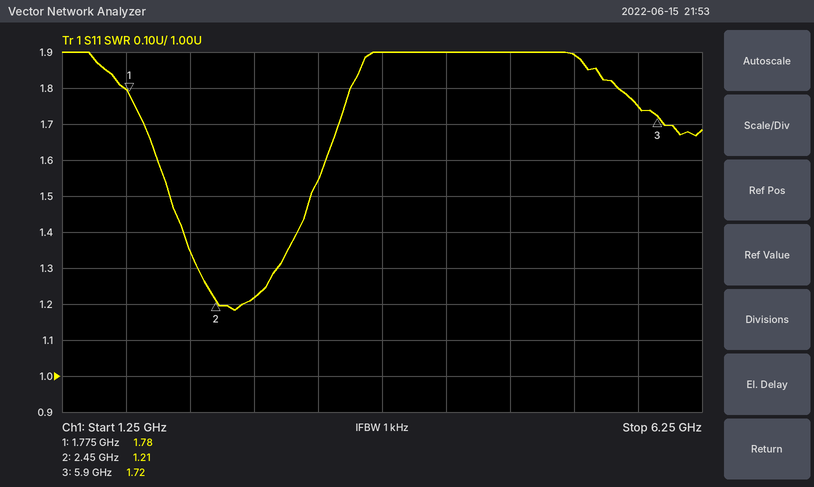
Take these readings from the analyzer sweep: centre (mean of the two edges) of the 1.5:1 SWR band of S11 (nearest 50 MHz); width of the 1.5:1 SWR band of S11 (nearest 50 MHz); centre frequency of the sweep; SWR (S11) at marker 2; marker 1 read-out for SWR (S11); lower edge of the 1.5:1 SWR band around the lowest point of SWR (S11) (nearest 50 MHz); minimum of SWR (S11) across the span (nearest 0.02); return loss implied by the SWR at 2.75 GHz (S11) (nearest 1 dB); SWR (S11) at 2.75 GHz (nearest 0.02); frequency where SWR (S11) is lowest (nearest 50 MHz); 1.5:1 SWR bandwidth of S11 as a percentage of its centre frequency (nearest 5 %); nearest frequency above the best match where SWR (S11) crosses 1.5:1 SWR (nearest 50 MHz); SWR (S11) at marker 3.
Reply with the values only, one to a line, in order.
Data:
2.65 GHz
1.10 GHz
3.75 GHz
1.21
1.78
2.10 GHz
1.18
20 dB
1.22
2.60 GHz
40 %
3.20 GHz
1.72
